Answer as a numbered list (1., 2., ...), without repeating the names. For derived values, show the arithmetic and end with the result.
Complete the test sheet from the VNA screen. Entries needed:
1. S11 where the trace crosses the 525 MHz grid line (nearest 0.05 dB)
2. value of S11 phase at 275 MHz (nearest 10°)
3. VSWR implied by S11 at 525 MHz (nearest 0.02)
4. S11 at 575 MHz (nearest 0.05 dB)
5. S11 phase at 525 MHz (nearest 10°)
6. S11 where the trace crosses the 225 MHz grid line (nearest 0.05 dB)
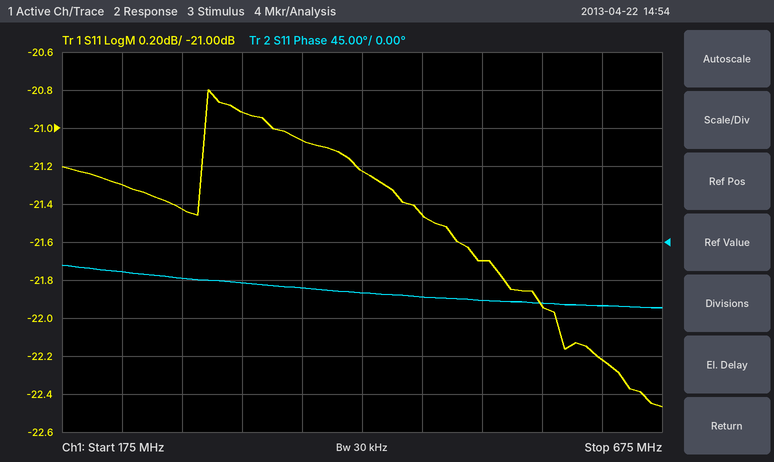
1. -21.70 dB
2. -40°
3. |Γ| = 10^(-21.7/20) = 0.0822; VSWR = (1 + 0.0822)/(1 − 0.0822) ≈ 1.18
4. -21.95 dB
5. -70°
6. -21.30 dB
